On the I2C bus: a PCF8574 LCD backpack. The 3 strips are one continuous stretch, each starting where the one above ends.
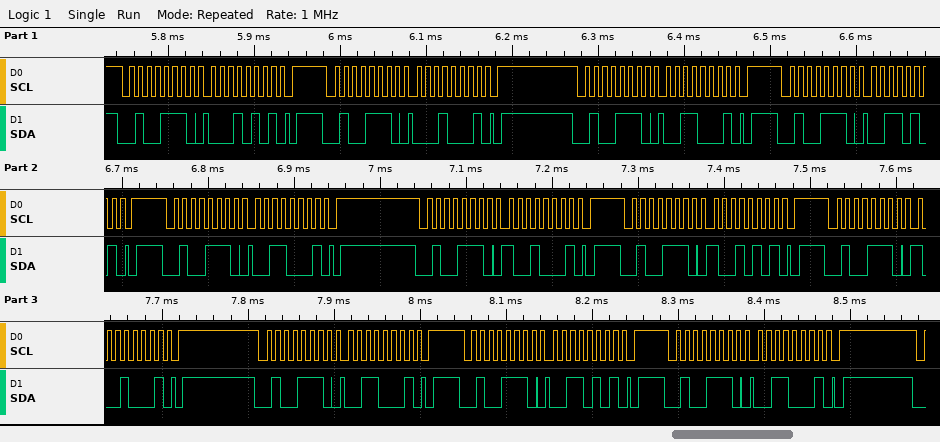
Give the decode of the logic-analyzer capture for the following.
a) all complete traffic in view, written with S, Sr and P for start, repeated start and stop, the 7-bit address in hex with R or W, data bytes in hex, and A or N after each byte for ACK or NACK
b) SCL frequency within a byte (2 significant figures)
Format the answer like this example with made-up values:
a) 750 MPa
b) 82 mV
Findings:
a) S 27W A 15 A P S 27W A 11 A P S 27W A 31 A P S 27W A 35 A P S 27W A 31 A P S 27W A 91 A P S 27W A 95 A P S 27W A 91 A P S 27W A 31 A P S 27W A 35 A P S 27W A 31 A P
b) 100 kHz
